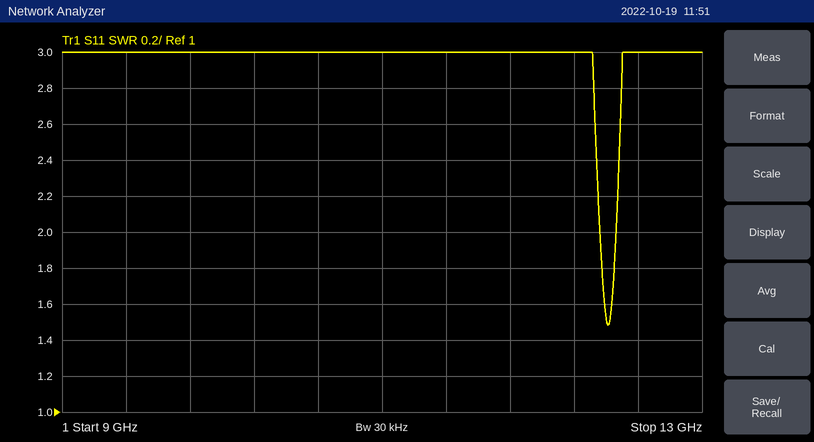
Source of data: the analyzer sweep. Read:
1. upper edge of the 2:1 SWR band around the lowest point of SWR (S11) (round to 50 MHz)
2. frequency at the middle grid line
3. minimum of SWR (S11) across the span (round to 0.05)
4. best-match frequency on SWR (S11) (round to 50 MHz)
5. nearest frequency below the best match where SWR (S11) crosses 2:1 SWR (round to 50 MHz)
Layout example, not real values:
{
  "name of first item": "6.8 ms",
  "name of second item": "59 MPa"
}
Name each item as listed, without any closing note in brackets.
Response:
{
  "upper edge of the 2:1 SWR band around the lowest point of SWR (S11)": "12.45 GHz",
  "frequency at the middle grid line": "11 GHz",
  "minimum of SWR (S11) across the span": "1.50",
  "best-match frequency on SWR (S11)": "12.40 GHz",
  "nearest frequency below the best match where SWR (S11) crosses 2:1 SWR": "12.35 GHz"
}
